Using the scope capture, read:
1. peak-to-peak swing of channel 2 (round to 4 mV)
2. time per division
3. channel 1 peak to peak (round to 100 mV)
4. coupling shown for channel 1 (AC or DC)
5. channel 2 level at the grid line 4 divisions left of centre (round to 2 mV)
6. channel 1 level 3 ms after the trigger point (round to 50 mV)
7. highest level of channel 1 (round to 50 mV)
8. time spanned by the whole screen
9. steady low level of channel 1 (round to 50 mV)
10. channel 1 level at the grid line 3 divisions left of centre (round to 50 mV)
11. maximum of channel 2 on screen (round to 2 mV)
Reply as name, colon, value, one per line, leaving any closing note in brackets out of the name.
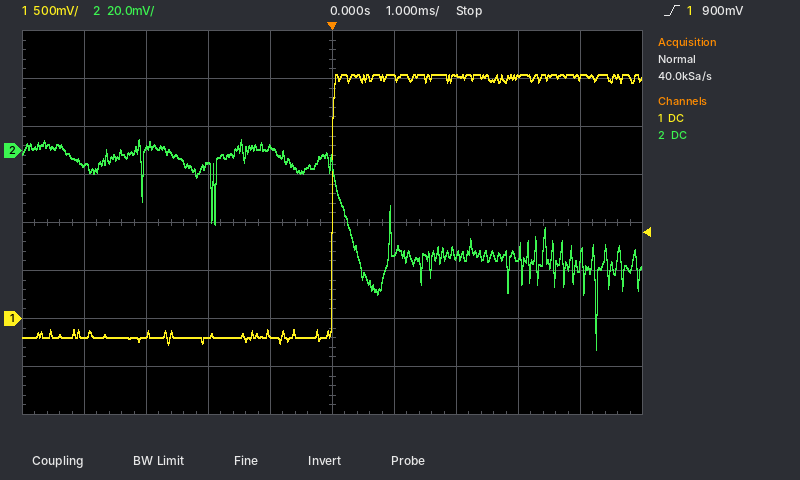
peak-to-peak swing of channel 2: 88 mV
time per division: 1 ms
channel 1 peak to peak: 2.80 V
coupling shown for channel 1: DC
channel 2 level at the grid line 4 divisions left of centre: -6 mV
channel 1 level 3 ms after the trigger point: 2.50 V
highest level of channel 1: 2.55 V
time spanned by the whole screen: 10 ms
steady low level of channel 1: -200 mV
channel 1 level at the grid line 3 divisions left of centre: -150 mV
maximum of channel 2 on screen: 4 mV
